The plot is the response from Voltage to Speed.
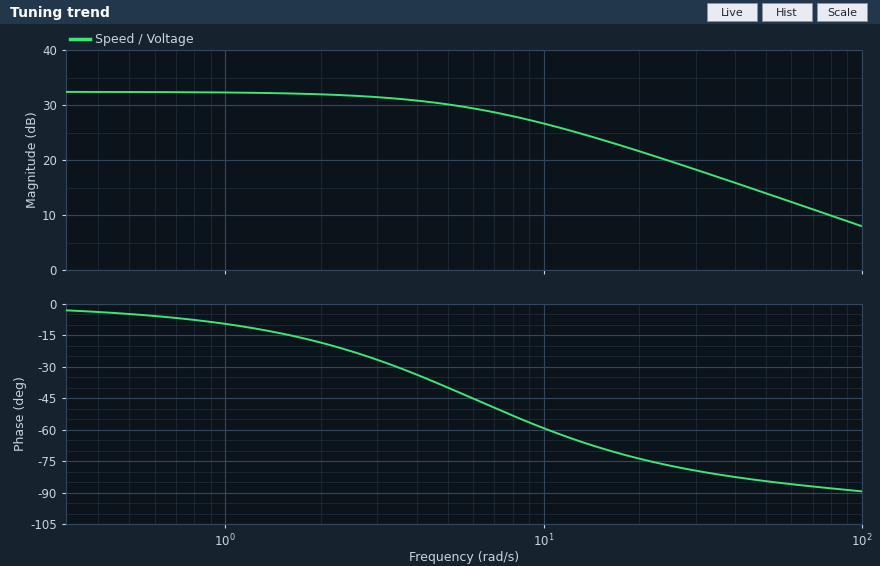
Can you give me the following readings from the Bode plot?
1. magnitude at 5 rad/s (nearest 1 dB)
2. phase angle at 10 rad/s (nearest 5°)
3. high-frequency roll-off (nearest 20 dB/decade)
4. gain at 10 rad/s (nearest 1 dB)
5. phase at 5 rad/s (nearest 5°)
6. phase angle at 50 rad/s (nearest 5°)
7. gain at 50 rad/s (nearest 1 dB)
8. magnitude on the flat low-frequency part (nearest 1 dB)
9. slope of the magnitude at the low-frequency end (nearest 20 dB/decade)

30 dB
-60°
-20 dB/decade
27 dB
-40°
-85°
14 dB
32 dB
0 dB/decade
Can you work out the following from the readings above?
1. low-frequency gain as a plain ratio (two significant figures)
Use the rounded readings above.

40
